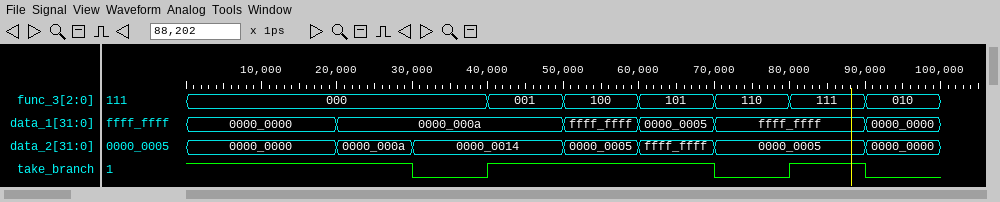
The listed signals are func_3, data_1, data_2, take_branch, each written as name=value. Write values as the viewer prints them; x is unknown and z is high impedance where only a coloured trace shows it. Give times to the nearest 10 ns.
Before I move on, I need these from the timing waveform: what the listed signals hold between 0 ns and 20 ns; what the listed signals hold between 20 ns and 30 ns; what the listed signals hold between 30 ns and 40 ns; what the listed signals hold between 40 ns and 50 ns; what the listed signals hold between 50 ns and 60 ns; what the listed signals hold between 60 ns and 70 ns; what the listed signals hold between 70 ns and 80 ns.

func_3=000, data_1=0000_0000, data_2=0000_0000, take_branch=1
func_3=000, data_1=0000_000a, data_2=0000_000a, take_branch=1
func_3=000, data_1=0000_000a, data_2=0000_0014, take_branch=0
func_3=001, data_1=0000_000a, data_2=0000_0014, take_branch=1
func_3=100, data_1=ffff_ffff, data_2=0000_0005, take_branch=1
func_3=101, data_1=0000_0005, data_2=ffff_ffff, take_branch=1
func_3=110, data_1=ffff_ffff, data_2=0000_0005, take_branch=0
